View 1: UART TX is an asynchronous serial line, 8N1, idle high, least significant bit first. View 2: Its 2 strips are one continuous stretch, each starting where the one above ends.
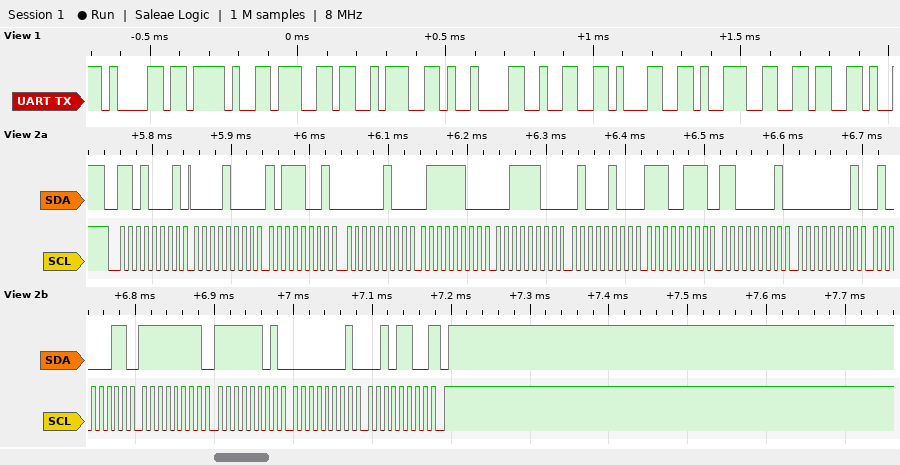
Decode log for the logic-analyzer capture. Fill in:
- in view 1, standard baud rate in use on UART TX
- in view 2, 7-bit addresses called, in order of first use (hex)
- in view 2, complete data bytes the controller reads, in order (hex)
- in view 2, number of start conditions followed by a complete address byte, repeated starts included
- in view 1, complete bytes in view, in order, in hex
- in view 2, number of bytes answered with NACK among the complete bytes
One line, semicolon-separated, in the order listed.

38400 baud; 0x68; 08 B9 04 7C 3C 44 E7 C1 01 43 FF FD 01 2C; 1; 0x61 0x2F 0x67 0x3A 0x09 0x32 0x31 0x39 0x36; 1
